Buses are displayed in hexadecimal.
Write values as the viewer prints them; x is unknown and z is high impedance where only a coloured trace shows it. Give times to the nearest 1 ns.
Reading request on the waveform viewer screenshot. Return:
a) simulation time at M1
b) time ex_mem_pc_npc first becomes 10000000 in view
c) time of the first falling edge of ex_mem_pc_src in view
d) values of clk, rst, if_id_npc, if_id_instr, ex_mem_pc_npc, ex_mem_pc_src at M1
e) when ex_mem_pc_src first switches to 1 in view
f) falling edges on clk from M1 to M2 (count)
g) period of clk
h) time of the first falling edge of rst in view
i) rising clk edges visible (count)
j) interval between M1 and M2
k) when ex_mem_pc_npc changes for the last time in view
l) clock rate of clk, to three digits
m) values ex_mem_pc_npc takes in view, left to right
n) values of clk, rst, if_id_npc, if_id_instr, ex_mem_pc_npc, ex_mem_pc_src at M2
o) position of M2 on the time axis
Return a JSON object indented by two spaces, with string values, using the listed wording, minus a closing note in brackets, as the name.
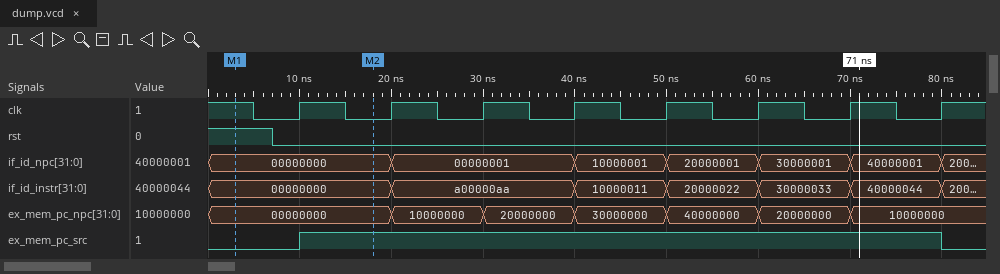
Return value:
{
  "simulation time at M1": "3 ns",
  "time ex_mem_pc_npc first becomes 10000000 in view": "20 ns",
  "time of the first falling edge of ex_mem_pc_src in view": "80 ns",
  "values of clk, rst, if_id_npc, if_id_instr, ex_mem_pc_npc, ex_mem_pc_src at M1": "clk=1, rst=1, if_id_npc=00000000, if_id_instr=00000000, ex_mem_pc_npc=00000000, ex_mem_pc_src=0",
  "when ex_mem_pc_src first switches to 1 in view": "10 ns",
  "falling edges on clk from M1 to M2": "2",
  "period of clk": "10 ns",
  "time of the first falling edge of rst in view": "7 ns",
  "rising clk edges visible": "8",
  "interval between M1 and M2": "15 ns",
  "when ex_mem_pc_npc changes for the last time in view": "70 ns",
  "clock rate of clk, to three digits": "100 MHz",
  "values ex_mem_pc_npc takes in view, left to right": "00000000, 10000000, 20000000, 30000000, 40000000, 20000000, 10000000",
  "values of clk, rst, if_id_npc, if_id_instr, ex_mem_pc_npc, ex_mem_pc_src at M2": "clk=0, rst=0, if_id_npc=00000000, if_id_instr=00000000, ex_mem_pc_npc=00000000, ex_mem_pc_src=1",
  "position of M2 on the time axis": "18 ns"
}
